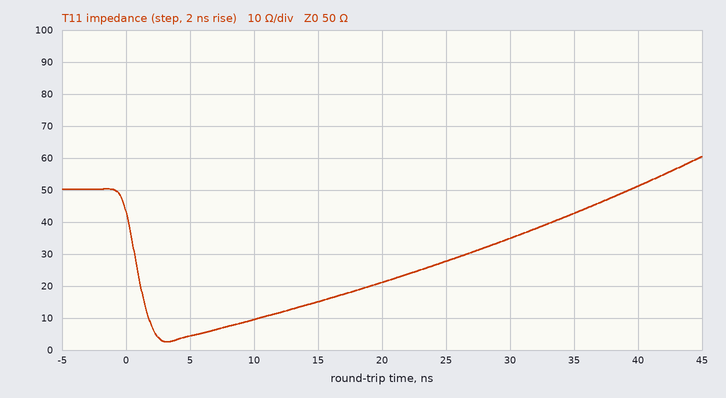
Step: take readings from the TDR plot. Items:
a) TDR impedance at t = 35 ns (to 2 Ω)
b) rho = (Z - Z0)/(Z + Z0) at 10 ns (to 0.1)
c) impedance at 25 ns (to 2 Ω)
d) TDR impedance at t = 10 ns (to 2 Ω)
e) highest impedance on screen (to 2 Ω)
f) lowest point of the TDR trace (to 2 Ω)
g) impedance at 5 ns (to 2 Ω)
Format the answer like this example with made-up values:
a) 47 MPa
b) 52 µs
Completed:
a) 42 Ω
b) -0.7
c) 28 Ω
d) 10 Ω
e) 60 Ω
f) 2 Ω
g) 4 Ω
